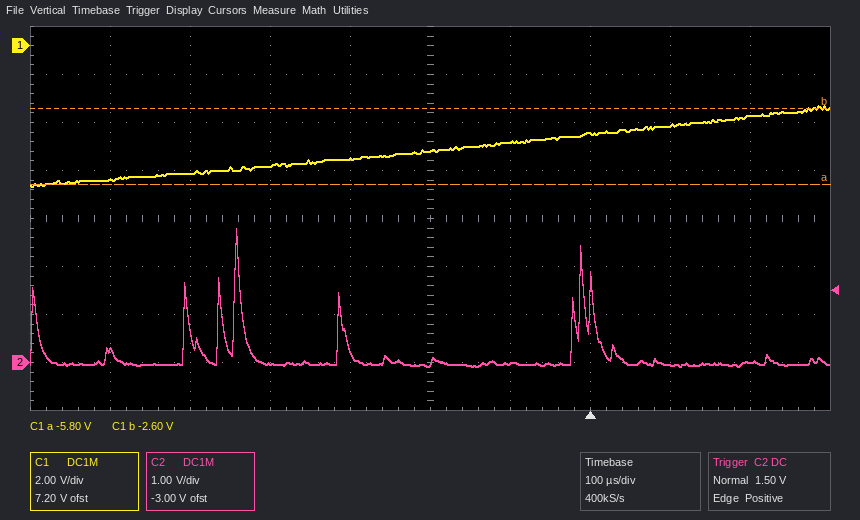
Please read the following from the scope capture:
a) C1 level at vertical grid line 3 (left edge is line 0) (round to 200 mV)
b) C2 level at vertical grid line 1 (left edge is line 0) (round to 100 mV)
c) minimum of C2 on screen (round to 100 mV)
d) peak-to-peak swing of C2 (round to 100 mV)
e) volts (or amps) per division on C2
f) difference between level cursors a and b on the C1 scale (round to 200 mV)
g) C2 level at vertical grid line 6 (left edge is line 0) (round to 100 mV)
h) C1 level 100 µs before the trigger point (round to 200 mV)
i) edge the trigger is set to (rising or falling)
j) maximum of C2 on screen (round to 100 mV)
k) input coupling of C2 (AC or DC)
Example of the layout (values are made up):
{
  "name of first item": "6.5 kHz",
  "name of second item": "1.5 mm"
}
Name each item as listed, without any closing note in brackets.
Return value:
{
  "C1 level at vertical grid line 3 (left edge is line 0)": "-5.0 V",
  "C2 level at vertical grid line 1 (left edge is line 0)": "200 mV",
  "minimum of C2 on screen": "-100 mV",
  "peak-to-peak swing of C2": "2.9 V",
  "volts (or amps) per division on C2": "1 V",
  "difference between level cursors a and b on the C1 scale": "3.2 V",
  "C2 level at vertical grid line 6 (left edge is line 0)": "0.0 V",
  "C1 level 100 µs before the trigger point": "-4.0 V",
  "edge the trigger is set to": "rising",
  "maximum of C2 on screen": "2.8 V",
  "input coupling of C2": "DC"
}
